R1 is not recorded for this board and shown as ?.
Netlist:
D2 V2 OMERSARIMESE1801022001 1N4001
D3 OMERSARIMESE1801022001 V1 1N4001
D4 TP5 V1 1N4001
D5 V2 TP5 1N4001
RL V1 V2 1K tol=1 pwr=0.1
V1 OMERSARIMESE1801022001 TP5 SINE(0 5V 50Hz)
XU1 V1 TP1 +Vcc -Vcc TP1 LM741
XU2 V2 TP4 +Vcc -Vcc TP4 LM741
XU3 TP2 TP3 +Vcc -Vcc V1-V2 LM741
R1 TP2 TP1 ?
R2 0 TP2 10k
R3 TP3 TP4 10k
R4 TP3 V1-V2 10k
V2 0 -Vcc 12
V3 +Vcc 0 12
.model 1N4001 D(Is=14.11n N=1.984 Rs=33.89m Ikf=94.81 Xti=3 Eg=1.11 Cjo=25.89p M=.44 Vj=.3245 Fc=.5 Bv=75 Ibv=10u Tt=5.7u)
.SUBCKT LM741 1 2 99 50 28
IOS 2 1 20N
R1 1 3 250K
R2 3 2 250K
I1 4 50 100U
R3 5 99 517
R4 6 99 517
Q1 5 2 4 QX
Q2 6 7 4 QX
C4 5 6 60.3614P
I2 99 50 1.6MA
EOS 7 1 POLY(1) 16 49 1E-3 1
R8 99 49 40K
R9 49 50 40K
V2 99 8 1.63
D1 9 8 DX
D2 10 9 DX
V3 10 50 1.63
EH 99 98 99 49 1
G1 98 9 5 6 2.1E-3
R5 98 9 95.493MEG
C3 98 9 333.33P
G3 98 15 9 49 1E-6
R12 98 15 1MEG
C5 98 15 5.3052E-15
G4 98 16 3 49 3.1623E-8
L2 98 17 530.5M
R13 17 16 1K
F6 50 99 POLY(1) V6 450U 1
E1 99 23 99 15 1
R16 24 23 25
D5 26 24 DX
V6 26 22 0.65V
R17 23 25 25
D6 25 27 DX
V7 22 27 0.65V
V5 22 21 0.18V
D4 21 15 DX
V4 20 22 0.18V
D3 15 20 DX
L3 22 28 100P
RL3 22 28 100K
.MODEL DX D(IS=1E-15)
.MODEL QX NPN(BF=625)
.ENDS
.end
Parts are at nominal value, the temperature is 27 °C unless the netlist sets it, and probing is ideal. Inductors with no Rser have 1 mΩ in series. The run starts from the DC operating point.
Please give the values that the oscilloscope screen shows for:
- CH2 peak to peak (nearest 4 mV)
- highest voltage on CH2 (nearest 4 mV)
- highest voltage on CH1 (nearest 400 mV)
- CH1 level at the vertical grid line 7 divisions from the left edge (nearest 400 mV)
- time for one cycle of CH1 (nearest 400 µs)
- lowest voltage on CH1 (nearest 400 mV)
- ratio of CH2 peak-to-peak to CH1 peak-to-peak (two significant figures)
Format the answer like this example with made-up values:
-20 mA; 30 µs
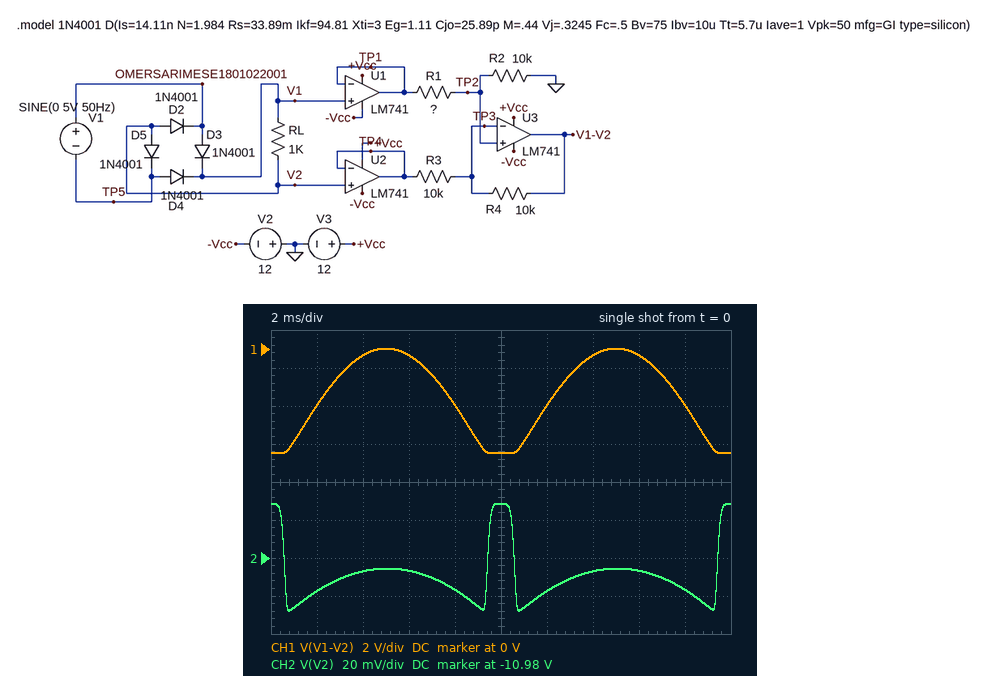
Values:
56 mV; -10.952 V; 0 V; -400 mV; 10.0 ms; -5.6 V; 0.010
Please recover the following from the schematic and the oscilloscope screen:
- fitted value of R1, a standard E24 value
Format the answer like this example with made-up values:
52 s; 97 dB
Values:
3.3 kΩ
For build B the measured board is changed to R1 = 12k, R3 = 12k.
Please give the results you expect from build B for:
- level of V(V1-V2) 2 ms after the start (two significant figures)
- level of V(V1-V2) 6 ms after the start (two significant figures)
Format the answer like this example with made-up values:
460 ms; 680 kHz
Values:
1.4 V; 2.9 V
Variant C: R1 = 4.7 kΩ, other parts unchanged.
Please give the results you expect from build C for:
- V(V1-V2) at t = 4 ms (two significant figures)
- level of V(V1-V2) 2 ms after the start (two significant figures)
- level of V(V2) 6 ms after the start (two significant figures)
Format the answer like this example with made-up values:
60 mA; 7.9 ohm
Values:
740 mV; -1.6 V; -11 V
